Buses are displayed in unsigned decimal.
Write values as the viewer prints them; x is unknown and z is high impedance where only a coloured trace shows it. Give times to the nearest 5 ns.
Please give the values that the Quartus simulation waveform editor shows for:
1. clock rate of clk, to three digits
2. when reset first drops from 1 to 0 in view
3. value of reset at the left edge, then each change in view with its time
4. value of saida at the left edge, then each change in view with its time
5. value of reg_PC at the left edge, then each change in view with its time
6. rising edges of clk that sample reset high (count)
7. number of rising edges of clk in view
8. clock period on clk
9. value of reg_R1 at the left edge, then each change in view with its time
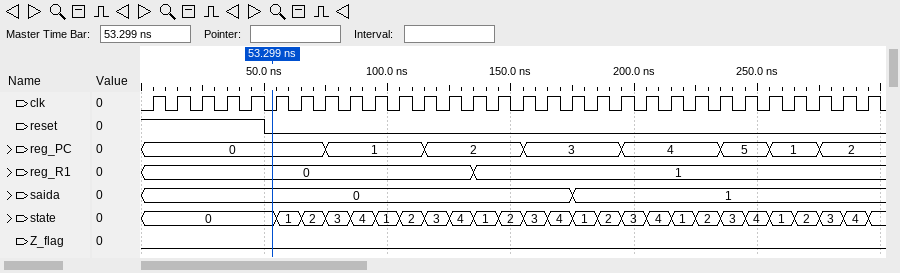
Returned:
100 MHz
50 ns
1, 0 at 50 ns
0, 1 at 175 ns
0, 1 at 75 ns, 2 at 115 ns, 3 at 155 ns, 4 at 195 ns, 5 at 235 ns, 1 at 255 ns, 2 at 275 ns
5
30
10 ns
0, 1 at 135 ns
